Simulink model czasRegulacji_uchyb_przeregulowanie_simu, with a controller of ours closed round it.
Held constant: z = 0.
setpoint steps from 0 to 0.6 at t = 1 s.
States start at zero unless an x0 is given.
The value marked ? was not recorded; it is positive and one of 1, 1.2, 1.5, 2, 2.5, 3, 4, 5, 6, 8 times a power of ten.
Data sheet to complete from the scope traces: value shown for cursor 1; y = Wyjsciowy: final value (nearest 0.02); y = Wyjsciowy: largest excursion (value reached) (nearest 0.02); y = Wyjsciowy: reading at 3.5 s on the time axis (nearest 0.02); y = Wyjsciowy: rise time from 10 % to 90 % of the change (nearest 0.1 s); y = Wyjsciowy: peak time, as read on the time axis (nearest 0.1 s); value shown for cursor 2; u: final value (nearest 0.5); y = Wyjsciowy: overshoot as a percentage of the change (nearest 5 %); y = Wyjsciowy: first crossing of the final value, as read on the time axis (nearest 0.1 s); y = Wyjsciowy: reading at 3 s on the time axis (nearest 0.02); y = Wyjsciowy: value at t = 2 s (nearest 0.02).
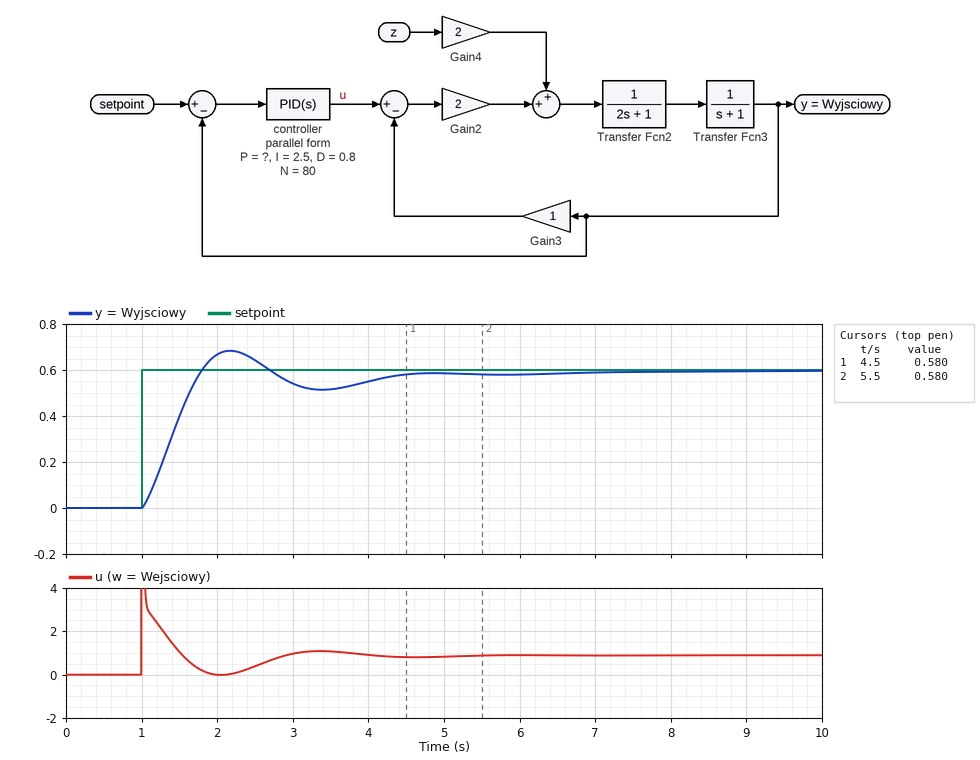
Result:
0.580
0.60
0.68
0.52
0.6 s
2.2 s
0.580
1.0
15 %
1.8 s
0.54
0.66
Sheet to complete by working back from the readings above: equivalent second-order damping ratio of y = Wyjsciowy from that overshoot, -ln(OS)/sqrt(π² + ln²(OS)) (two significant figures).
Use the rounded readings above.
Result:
0.52
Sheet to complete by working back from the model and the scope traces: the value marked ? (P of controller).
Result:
6
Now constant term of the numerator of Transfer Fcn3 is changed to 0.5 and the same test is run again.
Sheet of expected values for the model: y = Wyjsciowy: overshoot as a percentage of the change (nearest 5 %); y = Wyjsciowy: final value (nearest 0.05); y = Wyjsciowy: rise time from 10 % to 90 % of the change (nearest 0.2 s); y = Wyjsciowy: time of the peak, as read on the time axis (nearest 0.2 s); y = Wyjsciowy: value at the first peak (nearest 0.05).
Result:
10 %
0.60
1.0 s
2.8 s
0.65
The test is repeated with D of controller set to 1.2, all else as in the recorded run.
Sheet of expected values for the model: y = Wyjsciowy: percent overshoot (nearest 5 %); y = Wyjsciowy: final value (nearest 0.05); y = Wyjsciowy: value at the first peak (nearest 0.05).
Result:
10 %
0.60
0.65
